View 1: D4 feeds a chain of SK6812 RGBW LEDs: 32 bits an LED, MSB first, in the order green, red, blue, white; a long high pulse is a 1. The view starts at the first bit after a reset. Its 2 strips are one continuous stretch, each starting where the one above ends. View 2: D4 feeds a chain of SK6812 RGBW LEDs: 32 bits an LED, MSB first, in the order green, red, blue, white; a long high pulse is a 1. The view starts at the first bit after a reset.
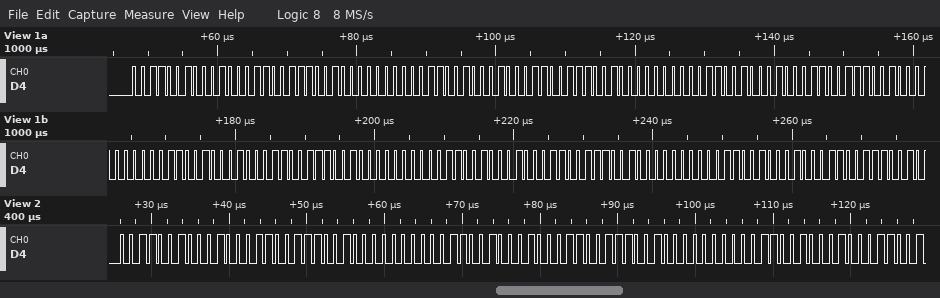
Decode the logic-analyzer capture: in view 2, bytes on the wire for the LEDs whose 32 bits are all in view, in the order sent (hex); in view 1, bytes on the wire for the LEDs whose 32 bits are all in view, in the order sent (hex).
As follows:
32 23 39 00 32 23 39 00
32 23 39 00 32 23 39 00 32 23 39 00 32 23 39 00 32 23 39 00
